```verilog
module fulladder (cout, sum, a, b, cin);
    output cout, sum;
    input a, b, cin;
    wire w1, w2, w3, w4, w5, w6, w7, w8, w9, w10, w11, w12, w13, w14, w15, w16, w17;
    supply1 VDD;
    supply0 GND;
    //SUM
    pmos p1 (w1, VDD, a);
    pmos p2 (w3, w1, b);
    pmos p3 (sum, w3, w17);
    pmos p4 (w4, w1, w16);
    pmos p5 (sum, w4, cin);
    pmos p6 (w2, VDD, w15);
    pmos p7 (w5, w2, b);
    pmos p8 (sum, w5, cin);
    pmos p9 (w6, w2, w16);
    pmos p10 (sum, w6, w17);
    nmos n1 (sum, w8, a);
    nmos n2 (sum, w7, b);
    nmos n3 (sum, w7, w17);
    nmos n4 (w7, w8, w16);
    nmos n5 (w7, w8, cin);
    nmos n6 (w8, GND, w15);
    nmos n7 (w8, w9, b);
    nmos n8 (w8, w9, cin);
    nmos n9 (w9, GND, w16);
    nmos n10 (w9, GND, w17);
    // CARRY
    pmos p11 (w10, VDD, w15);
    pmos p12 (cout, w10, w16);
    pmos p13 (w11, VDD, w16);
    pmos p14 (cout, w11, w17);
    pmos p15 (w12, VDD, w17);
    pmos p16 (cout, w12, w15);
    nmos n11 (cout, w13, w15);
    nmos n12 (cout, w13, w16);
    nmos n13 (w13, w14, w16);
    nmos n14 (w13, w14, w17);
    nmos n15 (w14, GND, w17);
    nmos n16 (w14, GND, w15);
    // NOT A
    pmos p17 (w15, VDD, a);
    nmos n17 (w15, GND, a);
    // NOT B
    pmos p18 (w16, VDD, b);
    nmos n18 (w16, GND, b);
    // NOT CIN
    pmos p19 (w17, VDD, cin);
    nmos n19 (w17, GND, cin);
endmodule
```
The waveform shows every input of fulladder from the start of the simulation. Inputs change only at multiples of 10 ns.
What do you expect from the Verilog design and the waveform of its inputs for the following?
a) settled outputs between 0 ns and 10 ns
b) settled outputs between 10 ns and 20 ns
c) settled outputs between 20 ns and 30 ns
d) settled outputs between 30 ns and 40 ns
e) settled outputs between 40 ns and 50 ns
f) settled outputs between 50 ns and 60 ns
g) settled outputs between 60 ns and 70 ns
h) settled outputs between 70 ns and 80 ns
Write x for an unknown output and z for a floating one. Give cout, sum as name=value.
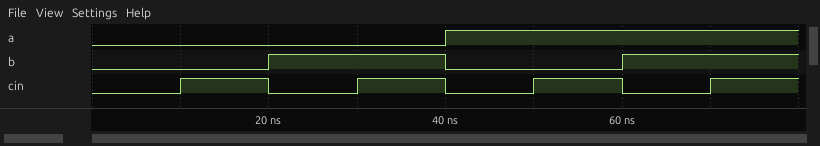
cout=0, sum=0
cout=0, sum=1
cout=0, sum=1
cout=1, sum=0
cout=0, sum=1
cout=1, sum=0
cout=1, sum=0
cout=1, sum=1
